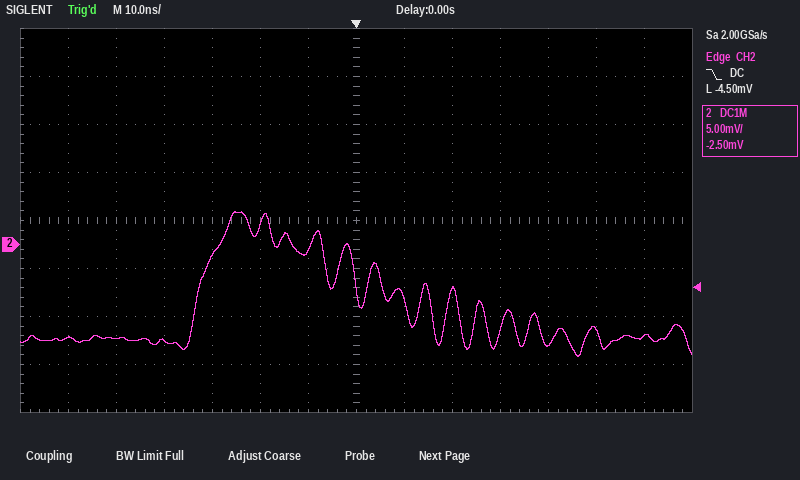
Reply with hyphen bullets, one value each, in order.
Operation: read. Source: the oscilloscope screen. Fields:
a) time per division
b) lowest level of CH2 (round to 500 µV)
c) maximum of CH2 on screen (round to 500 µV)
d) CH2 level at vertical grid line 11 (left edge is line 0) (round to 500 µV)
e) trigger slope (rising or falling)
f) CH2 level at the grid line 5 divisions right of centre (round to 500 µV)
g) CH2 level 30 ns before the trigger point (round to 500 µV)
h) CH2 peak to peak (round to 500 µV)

- 10 ns
- -11.5 mV
- 3.5 mV
- -10.5 mV
- falling
- -9.0 mV
- -1.0 mV
- 15.0 mV
